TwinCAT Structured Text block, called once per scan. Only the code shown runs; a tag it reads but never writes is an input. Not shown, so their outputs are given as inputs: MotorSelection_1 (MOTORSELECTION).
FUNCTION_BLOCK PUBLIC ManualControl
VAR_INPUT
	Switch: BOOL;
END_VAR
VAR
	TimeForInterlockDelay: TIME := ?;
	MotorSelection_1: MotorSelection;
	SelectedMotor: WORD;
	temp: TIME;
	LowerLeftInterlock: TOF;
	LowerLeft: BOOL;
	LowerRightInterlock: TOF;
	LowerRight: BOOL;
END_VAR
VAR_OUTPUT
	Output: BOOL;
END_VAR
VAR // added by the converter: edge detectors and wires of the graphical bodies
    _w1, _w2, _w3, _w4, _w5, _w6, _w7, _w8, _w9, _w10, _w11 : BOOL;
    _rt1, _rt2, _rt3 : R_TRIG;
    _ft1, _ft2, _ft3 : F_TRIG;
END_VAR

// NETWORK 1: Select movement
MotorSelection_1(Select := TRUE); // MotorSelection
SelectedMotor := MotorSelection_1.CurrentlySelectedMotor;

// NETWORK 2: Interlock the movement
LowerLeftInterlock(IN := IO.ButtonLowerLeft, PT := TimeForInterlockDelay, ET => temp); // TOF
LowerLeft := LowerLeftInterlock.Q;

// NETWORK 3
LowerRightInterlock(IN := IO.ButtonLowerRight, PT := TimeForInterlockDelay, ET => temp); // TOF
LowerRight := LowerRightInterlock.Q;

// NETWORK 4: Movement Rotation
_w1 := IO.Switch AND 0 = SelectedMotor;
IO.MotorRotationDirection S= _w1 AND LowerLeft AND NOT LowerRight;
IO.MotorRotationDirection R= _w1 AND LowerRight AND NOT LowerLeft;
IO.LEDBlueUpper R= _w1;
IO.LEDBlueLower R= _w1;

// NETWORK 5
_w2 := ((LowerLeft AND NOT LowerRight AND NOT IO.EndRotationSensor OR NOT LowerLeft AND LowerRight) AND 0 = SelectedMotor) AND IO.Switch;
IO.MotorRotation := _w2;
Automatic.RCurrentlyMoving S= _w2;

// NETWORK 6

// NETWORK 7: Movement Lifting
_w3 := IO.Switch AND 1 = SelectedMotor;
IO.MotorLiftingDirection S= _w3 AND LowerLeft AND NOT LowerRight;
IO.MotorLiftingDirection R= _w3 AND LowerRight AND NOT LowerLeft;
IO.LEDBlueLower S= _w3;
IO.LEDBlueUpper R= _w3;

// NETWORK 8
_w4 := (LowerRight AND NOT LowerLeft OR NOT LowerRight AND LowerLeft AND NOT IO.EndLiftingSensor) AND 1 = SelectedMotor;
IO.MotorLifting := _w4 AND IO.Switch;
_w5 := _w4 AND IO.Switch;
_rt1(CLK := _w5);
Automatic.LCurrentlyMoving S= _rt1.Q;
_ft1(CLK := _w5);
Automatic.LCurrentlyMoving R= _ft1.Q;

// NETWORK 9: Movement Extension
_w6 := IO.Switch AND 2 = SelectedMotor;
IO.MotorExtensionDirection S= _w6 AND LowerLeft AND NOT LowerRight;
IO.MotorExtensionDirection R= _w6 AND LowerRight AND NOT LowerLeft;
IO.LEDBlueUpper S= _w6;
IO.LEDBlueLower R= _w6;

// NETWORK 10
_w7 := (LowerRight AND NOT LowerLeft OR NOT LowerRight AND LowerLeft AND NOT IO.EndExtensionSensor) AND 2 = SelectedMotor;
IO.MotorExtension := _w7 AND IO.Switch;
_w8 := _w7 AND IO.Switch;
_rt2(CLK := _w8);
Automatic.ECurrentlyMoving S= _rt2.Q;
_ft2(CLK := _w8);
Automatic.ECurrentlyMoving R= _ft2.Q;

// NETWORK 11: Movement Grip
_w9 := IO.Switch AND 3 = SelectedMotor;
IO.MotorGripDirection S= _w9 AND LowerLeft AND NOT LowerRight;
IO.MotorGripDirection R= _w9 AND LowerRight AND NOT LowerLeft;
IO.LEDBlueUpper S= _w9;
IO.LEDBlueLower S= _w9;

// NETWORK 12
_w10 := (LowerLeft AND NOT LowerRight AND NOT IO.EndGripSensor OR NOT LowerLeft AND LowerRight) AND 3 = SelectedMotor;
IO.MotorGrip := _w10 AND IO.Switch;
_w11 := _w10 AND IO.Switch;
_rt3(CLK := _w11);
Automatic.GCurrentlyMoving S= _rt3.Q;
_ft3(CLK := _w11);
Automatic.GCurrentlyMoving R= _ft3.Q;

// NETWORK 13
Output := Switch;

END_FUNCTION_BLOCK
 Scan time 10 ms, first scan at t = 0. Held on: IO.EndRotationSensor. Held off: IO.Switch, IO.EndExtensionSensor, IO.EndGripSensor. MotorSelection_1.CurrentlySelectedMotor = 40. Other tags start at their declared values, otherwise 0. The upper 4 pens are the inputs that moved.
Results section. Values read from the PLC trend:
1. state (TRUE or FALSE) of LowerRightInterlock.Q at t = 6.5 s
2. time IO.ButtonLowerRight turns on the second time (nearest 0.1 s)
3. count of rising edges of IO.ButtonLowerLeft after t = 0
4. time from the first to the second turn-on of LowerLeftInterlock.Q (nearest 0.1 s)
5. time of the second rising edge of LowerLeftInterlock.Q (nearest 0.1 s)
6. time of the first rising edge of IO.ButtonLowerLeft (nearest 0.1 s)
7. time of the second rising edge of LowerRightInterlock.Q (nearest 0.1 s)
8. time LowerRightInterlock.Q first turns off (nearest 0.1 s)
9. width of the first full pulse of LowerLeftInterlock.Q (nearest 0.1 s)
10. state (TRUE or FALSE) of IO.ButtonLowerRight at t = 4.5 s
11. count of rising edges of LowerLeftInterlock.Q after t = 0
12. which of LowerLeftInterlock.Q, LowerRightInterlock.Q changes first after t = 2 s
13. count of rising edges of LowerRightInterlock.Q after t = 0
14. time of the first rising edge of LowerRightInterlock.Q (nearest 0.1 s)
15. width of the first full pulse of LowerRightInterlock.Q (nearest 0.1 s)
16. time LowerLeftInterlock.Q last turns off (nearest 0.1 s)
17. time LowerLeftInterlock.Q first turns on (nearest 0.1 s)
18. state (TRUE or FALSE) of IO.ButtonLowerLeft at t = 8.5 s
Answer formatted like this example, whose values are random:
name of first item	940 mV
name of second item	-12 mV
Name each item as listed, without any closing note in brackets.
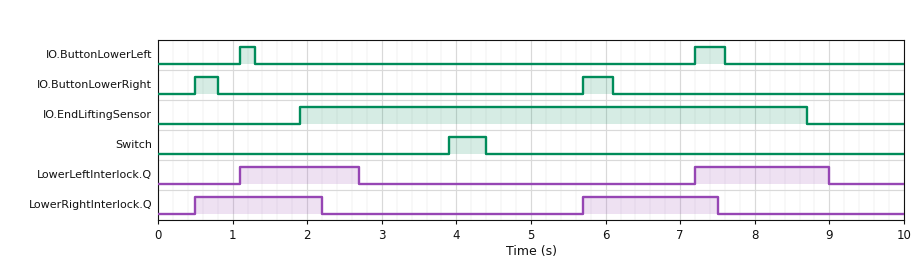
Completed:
state (TRUE or FALSE) of LowerRightInterlock.Q at t = 6.5 s	TRUE
time IO.ButtonLowerRight turns on the second time	5.7 s
count of rising edges of IO.ButtonLowerLeft after t = 0	2
time from the first to the second turn-on of LowerLeftInterlock.Q	6.1 s
time of the second rising edge of LowerLeftInterlock.Q	7.2 s
time of the first rising edge of IO.ButtonLowerLeft	1.1 s
time of the second rising edge of LowerRightInterlock.Q	5.7 s
time LowerRightInterlock.Q first turns off	2.2 s
width of the first full pulse of LowerLeftInterlock.Q	1.6 s
state (TRUE or FALSE) of IO.ButtonLowerRight at t = 4.5 s	FALSE
count of rising edges of LowerLeftInterlock.Q after t = 0	2
which of LowerLeftInterlock.Q, LowerRightInterlock.Q changes first after t = 2 s	LowerRightInterlock.Q
count of rising edges of LowerRightInterlock.Q after t = 0	2
time of the first rising edge of LowerRightInterlock.Q	0.5 s
width of the first full pulse of LowerRightInterlock.Q	1.7 s
time LowerLeftInterlock.Q last turns off	9.0 s
time LowerLeftInterlock.Q first turns on	1.1 s
state (TRUE or FALSE) of IO.ButtonLowerLeft at t = 8.5 s	FALSE
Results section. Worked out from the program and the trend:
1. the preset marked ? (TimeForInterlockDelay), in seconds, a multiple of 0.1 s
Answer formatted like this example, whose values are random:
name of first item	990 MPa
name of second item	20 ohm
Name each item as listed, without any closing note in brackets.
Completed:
the preset marked ? (TimeForInterlockDelay), in seconds, a multiple of 0.1 s	1.4 s
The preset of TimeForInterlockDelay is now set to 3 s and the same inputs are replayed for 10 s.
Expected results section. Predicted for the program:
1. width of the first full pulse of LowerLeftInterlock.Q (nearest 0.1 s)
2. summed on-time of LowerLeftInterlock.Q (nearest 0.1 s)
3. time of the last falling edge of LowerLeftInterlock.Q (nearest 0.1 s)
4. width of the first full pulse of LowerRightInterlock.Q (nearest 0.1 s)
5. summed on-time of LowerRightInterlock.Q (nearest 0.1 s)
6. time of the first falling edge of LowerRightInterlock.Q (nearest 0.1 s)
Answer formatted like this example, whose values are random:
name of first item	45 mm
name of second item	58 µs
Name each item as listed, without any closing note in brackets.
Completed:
width of the first full pulse of LowerLeftInterlock.Q	3.2 s
summed on-time of LowerLeftInterlock.Q	6.0 s
time of the last falling edge of LowerLeftInterlock.Q	4.3 s
width of the first full pulse of LowerRightInterlock.Q	3.3 s
summed on-time of LowerRightInterlock.Q	6.7 s
time of the first falling edge of LowerRightInterlock.Q	3.8 s
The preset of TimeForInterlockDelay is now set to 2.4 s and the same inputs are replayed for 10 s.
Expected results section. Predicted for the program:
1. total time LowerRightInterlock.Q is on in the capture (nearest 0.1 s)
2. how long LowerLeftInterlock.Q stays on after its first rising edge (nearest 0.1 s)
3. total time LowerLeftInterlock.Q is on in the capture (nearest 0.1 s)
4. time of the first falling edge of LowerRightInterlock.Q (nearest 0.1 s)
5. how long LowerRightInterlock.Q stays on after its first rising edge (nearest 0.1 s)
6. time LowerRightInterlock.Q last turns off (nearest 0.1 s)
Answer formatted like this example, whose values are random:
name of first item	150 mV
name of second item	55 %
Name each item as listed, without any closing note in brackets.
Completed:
total time LowerRightInterlock.Q is on in the capture	5.5 s
how long LowerLeftInterlock.Q stays on after its first rising edge	2.6 s
total time LowerLeftInterlock.Q is on in the capture	5.4 s
time of the first falling edge of LowerRightInterlock.Q	3.2 s
how long LowerRightInterlock.Q stays on after its first rising edge	2.7 s
time LowerRightInterlock.Q last turns off	8.5 s
